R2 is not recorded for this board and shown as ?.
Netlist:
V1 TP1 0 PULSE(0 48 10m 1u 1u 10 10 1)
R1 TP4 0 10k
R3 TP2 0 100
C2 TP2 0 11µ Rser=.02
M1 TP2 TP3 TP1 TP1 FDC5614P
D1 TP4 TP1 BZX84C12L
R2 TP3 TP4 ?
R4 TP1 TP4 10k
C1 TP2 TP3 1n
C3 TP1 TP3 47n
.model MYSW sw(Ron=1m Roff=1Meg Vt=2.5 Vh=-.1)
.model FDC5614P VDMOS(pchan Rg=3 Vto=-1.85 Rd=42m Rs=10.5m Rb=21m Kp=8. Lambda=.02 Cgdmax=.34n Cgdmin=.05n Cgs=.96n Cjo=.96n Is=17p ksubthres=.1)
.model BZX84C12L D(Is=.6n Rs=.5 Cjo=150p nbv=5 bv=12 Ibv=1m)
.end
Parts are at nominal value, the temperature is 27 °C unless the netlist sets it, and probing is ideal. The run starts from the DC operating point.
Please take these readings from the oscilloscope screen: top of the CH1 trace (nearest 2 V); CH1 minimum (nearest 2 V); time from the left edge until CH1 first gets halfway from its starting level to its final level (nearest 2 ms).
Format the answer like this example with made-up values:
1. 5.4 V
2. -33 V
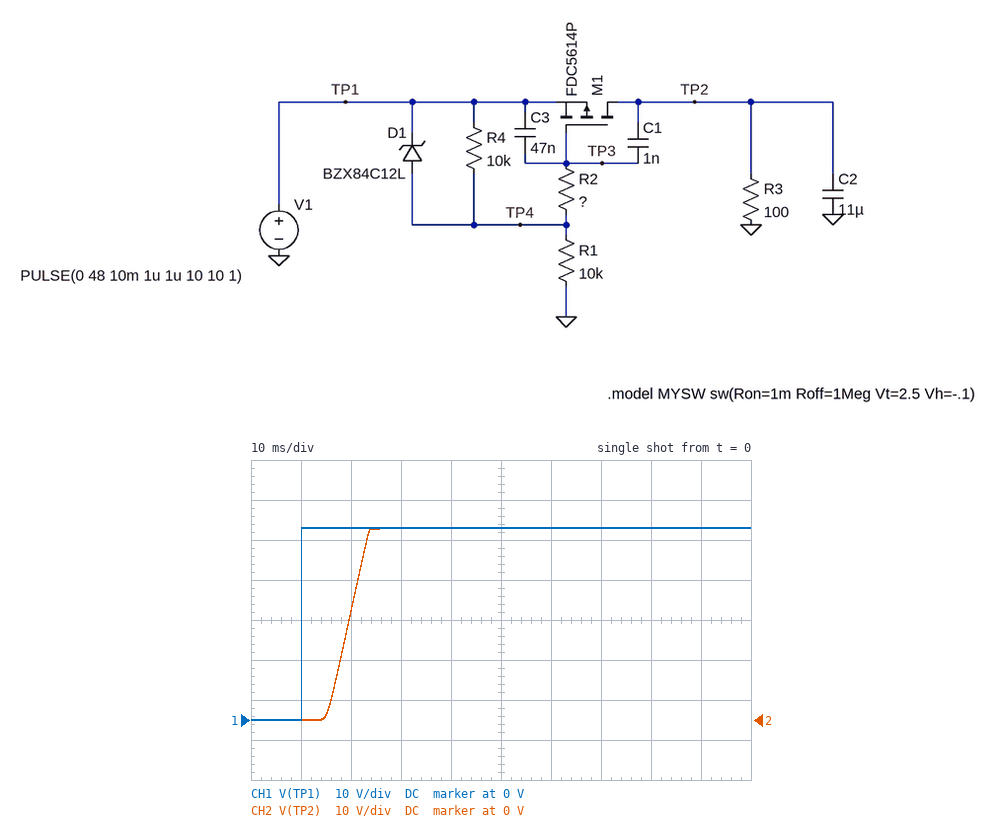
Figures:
1. 48 V
2. 0 V
3. 10 ms
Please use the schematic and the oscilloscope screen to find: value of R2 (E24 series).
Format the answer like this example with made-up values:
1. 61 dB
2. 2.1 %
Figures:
1. 1.3 MΩ
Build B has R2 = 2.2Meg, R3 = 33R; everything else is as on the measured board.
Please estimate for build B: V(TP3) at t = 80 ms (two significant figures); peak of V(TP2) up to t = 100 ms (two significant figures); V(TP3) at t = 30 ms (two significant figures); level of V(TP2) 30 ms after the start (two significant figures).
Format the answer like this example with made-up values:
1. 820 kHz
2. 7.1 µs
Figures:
1. 42 V
2. 48 V
3. 46 V
4. 31 V
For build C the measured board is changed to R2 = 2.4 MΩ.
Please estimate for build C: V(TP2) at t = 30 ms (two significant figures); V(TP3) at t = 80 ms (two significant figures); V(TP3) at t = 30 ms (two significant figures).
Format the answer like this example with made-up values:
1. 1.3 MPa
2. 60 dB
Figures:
1. 32 V
2. 43 V
3. 46 V
